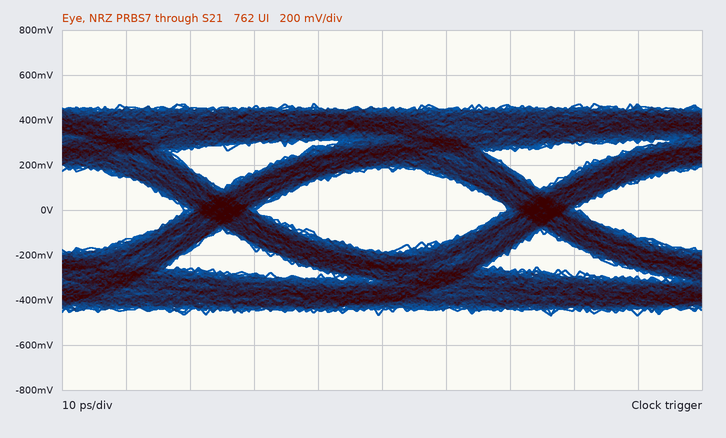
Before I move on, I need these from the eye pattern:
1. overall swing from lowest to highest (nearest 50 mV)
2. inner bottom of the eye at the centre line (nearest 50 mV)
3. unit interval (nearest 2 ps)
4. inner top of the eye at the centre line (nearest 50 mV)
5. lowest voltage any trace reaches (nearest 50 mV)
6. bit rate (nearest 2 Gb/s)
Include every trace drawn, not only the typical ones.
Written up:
950 mV
-200 mV
50 ps
200 mV
-450 mV
20 Gb/s
